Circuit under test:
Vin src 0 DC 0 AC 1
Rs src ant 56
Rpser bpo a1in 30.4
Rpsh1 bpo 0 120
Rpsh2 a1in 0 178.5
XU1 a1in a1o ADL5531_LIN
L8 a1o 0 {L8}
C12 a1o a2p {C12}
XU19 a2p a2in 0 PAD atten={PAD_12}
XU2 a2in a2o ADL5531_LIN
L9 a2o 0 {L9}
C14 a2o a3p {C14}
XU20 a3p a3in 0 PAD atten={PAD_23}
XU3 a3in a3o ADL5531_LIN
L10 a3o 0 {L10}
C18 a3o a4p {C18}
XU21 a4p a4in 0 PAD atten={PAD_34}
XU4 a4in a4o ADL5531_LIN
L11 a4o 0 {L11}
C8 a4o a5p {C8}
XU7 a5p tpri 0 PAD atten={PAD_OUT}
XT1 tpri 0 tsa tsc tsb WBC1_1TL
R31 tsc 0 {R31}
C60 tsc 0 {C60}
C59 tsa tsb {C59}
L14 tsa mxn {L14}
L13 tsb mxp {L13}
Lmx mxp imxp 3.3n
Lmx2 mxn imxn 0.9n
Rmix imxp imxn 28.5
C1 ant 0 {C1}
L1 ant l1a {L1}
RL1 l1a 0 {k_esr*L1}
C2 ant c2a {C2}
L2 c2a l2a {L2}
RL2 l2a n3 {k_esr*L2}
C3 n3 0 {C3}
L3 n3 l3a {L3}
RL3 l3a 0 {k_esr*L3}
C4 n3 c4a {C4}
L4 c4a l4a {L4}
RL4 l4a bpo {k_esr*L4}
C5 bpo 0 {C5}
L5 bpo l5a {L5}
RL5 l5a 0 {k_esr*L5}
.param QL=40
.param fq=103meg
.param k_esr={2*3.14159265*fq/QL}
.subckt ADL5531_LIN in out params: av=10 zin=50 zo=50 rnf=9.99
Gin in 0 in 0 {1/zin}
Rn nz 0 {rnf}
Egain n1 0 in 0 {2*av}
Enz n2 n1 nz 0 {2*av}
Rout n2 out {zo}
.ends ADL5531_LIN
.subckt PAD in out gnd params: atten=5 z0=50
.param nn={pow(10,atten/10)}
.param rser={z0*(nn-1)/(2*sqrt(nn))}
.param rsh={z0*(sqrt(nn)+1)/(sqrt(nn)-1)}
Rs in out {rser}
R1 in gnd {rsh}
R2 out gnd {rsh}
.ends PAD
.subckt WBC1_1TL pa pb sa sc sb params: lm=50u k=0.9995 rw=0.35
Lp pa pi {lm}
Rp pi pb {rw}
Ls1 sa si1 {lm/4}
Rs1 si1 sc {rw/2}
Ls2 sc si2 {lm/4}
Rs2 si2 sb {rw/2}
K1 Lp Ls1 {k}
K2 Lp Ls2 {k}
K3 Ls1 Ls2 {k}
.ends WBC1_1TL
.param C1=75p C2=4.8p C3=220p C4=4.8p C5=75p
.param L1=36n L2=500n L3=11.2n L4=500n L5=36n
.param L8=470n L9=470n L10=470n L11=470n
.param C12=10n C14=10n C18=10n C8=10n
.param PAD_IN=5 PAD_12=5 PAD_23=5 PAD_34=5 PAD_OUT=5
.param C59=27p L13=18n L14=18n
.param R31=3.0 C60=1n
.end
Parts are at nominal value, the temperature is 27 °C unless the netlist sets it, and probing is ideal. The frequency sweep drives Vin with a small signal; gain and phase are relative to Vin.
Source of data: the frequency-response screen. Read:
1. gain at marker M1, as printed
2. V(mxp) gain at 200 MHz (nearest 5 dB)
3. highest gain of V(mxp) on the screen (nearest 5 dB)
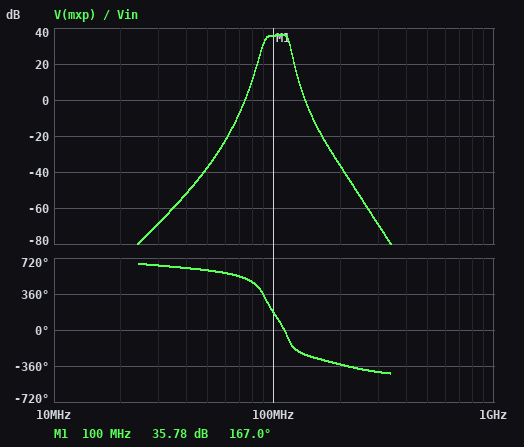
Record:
35.78 dB
-35 dB
35 dB
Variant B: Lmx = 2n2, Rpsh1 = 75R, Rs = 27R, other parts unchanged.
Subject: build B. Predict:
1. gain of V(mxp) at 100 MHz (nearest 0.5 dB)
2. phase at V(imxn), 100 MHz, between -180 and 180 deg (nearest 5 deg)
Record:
37.5 dB
-10 deg
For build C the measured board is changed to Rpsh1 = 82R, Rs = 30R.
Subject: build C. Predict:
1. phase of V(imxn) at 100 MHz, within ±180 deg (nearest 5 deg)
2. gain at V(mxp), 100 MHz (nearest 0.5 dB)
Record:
-10 deg
37.5 dB
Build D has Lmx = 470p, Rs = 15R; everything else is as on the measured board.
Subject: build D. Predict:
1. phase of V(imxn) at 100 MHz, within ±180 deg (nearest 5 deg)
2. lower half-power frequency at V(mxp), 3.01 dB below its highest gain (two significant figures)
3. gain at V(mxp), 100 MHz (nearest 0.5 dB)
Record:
-10 deg
92 MHz
39.5 dB
